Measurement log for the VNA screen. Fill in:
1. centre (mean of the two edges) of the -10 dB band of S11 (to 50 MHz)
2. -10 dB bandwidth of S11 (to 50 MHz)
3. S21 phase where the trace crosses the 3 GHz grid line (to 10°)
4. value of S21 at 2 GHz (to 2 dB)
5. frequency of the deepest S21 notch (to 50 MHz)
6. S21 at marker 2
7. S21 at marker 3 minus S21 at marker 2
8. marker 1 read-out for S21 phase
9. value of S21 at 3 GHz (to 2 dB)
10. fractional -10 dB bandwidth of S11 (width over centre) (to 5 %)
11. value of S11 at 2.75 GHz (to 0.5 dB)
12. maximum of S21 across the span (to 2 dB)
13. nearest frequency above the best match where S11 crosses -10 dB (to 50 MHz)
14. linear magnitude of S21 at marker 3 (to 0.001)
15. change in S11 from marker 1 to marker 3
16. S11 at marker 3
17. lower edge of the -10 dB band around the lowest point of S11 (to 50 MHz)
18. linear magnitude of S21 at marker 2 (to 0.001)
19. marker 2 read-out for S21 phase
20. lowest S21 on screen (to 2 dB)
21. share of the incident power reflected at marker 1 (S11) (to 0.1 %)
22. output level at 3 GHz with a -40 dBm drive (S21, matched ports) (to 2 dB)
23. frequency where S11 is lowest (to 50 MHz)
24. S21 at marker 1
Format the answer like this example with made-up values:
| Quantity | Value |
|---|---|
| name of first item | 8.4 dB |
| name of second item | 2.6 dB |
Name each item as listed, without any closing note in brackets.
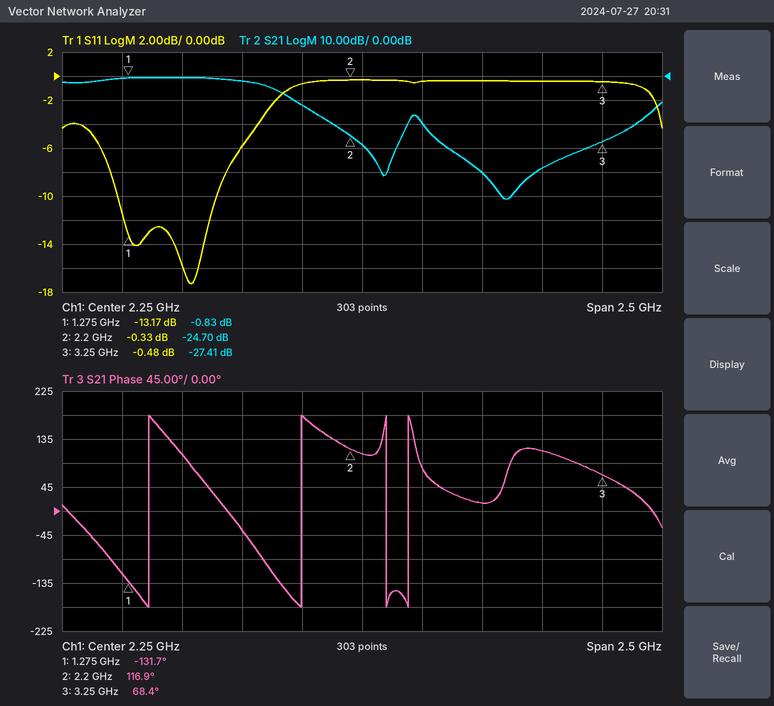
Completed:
| Quantity | Value |
|---|---|
| centre (mean of the two edges) of the -10 dB band of S11 | 1.45 GHz |
| -10 dB bandwidth of S11 | 400 MHz |
| S21 phase where the trace crosses the 3 GHz grid line | 110° |
| value of S21 at 2 GHz | -12 dB |
| frequency of the deepest S21 notch | 2.85 GHz |
| S21 at marker 2 | -24.70 dB |
| S21 at marker 3 minus S21 at marker 2 | -2.71 dB |
| marker 1 read-out for S21 phase | -131.7° |
| value of S21 at 3 GHz | -38 dB |
| fractional -10 dB bandwidth of S11 (width over centre) | 30 % |
| value of S11 at 2.75 GHz | -0.5 dB |
| maximum of S21 across the span | 0 dB |
| nearest frequency above the best match where S11 crosses -10 dB | 1.65 GHz |
| linear magnitude of S21 at marker 3 | 0.043 |
| change in S11 from marker 1 to marker 3 | 12.69 dB |
| S11 at marker 3 | -0.48 dB |
| lower edge of the -10 dB band around the lowest point of S11 | 1.25 GHz |
| linear magnitude of S21 at marker 2 | 0.058 |
| marker 2 read-out for S21 phase | 116.9° |
| lowest S21 on screen | -52 dB |
| share of the incident power reflected at marker 1 (S11) | 4.8 % |
| output level at 3 GHz with a -40 dBm drive (S21, matched ports) | -78 dBm |
| frequency where S11 is lowest | 1.55 GHz |
| S21 at marker 1 | -0.83 dB |
